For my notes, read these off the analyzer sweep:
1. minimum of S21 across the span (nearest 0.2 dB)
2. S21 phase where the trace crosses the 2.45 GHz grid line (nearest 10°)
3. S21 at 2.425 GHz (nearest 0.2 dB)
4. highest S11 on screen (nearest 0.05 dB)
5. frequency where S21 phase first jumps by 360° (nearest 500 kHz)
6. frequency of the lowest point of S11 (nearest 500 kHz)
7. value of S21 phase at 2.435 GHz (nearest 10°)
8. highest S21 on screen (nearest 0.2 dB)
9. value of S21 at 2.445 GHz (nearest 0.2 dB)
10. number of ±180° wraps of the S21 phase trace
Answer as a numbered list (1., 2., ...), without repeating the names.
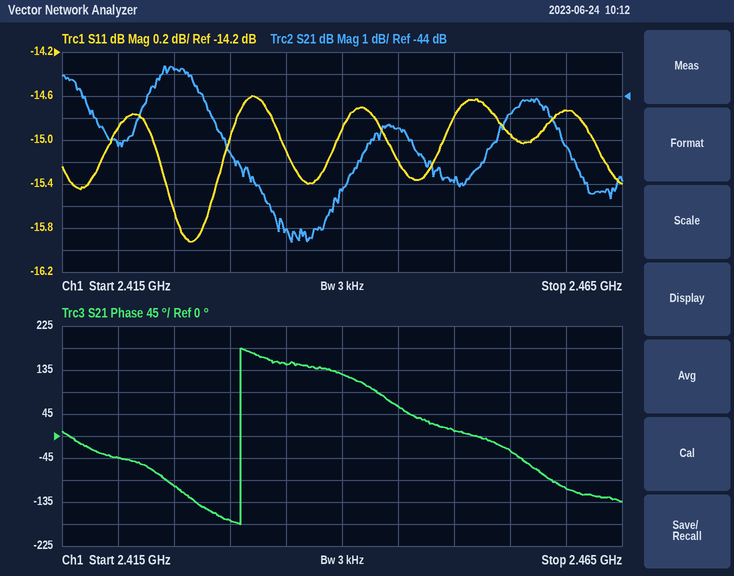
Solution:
1. -50.6 dB
2. 10°
3. -42.8 dB
4. -14.60 dB
5. 2.4310 GHz
6. 2.4265 GHz
7. 150°
8. -42.6 dB
9. -45.4 dB
10. 1
